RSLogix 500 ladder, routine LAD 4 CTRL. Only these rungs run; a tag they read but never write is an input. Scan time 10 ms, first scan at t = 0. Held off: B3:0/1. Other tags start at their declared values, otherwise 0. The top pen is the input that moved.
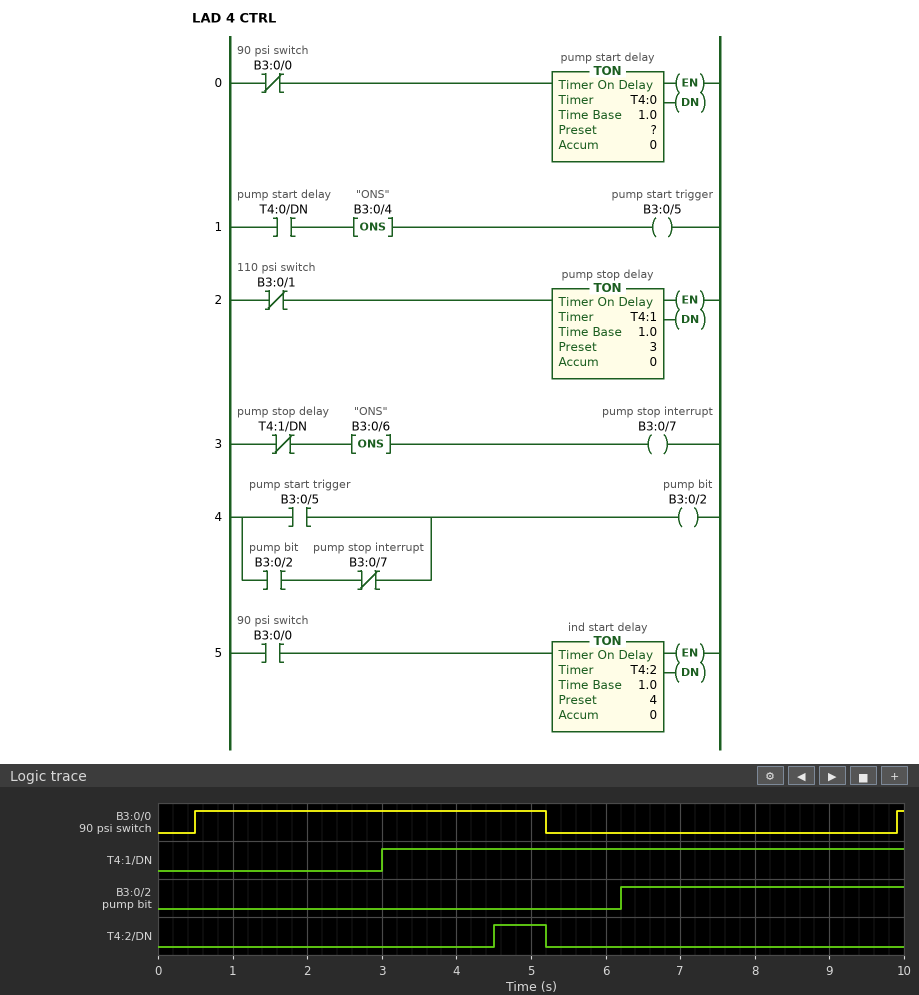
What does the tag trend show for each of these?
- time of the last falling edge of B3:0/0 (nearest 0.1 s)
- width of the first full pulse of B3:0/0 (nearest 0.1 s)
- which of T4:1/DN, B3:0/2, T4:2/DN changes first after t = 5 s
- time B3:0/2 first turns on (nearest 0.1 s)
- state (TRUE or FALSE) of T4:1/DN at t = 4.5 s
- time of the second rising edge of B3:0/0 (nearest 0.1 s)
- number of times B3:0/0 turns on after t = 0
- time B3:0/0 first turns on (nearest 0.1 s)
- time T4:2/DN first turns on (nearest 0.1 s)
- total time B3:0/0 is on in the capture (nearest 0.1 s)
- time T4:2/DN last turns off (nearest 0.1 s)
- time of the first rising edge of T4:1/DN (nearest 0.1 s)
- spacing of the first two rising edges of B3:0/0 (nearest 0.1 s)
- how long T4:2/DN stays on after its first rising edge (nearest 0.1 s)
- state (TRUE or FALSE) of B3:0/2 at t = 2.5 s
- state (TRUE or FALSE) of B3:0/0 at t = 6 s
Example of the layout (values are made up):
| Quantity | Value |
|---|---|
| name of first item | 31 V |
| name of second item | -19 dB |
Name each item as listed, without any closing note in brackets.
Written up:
| Quantity | Value |
|---|---|
| time of the last falling edge of B3:0/0 | 5.2 s |
| width of the first full pulse of B3:0/0 | 4.7 s |
| which of T4:1/DN, B3:0/2, T4:2/DN changes first after t = 5 s | T4:2/DN |
| time B3:0/2 first turns on | 6.2 s |
| state (TRUE or FALSE) of T4:1/DN at t = 4.5 s | TRUE |
| time of the second rising edge of B3:0/0 | 9.9 s |
| number of times B3:0/0 turns on after t = 0 | 2 |
| time B3:0/0 first turns on | 0.5 s |
| time T4:2/DN first turns on | 4.5 s |
| total time B3:0/0 is on in the capture | 4.8 s |
| time T4:2/DN last turns off | 5.2 s |
| time of the first rising edge of T4:1/DN | 3.0 s |
| spacing of the first two rising edges of B3:0/0 | 9.4 s |
| how long T4:2/DN stays on after its first rising edge | 0.7 s |
| state (TRUE or FALSE) of B3:0/2 at t = 2.5 s | FALSE |
| state (TRUE or FALSE) of B3:0/0 at t = 6 s | FALSE |
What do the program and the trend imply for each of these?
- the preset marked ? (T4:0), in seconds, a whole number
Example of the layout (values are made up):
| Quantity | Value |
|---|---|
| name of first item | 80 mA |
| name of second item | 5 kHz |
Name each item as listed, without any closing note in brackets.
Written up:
| Quantity | Value |
|---|---|
| the preset marked ? (T4:0), in seconds, a whole number | 1 s |
